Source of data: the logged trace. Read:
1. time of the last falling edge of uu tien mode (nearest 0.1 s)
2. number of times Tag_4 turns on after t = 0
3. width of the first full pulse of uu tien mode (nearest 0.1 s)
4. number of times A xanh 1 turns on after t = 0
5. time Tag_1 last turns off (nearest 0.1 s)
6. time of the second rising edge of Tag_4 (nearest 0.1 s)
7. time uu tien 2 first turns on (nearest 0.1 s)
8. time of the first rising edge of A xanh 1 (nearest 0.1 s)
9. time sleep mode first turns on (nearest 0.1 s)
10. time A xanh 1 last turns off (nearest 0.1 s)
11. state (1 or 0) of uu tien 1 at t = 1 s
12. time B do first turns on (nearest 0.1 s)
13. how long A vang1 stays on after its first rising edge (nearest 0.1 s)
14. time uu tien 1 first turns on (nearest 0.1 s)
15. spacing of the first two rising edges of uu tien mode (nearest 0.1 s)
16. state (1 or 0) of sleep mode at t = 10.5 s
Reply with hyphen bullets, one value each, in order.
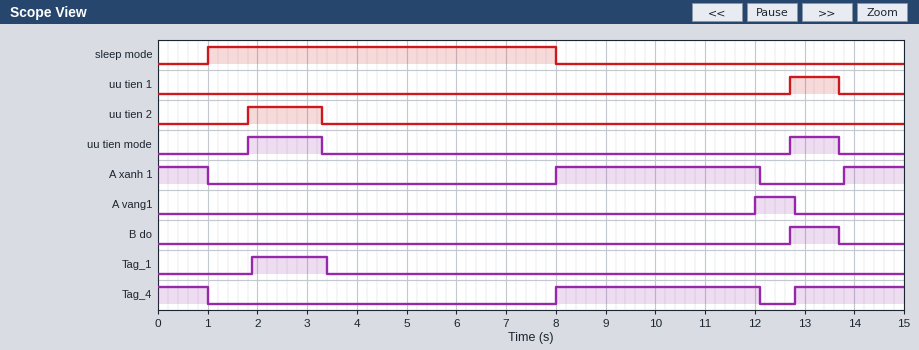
- 13.7 s
- 2
- 1.5 s
- 2
- 3.4 s
- 12.8 s
- 1.8 s
- 8.0 s
- 1.0 s
- 12.1 s
- 0
- 12.7 s
- 0.8 s
- 12.7 s
- 10.9 s
- 0
